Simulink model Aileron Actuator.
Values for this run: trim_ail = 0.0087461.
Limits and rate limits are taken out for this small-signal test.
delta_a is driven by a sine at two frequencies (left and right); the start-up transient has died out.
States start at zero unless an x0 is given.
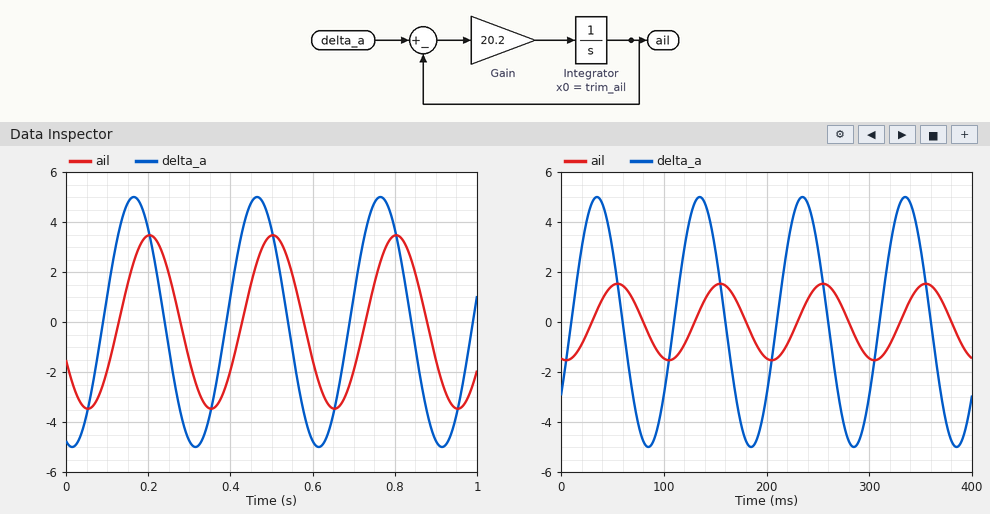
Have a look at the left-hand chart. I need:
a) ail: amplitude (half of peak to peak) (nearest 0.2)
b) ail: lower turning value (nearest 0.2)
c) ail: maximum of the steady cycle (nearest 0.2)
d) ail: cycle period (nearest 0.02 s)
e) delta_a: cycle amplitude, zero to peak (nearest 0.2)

3.4
-3.4
3.4
0.30 s
5.0
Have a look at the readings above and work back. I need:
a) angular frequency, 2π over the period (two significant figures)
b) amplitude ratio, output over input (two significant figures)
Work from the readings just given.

21 rad/s
0.68
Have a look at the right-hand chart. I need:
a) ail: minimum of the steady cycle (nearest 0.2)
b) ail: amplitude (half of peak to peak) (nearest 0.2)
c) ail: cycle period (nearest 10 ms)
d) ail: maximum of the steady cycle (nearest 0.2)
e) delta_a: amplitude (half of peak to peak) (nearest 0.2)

-1.6
1.6
100 ms
1.6
5.0
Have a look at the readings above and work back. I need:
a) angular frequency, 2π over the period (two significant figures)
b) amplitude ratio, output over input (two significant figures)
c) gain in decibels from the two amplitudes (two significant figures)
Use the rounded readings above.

0.063 rad/ms
0.32
-9.9 dB
